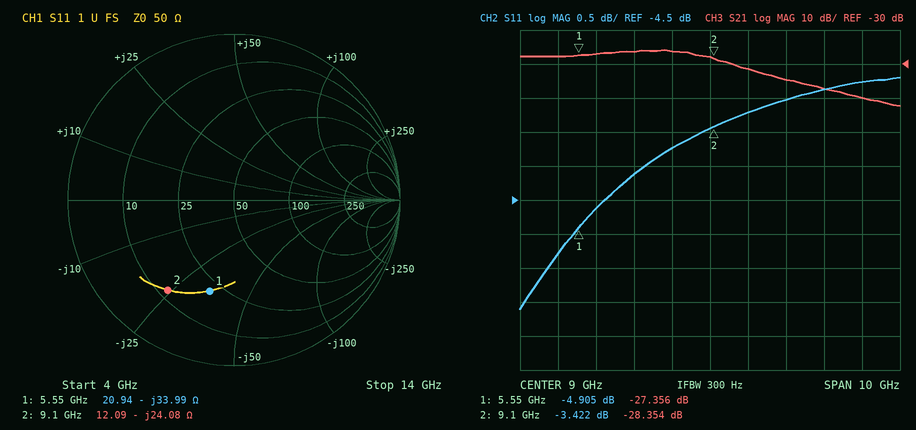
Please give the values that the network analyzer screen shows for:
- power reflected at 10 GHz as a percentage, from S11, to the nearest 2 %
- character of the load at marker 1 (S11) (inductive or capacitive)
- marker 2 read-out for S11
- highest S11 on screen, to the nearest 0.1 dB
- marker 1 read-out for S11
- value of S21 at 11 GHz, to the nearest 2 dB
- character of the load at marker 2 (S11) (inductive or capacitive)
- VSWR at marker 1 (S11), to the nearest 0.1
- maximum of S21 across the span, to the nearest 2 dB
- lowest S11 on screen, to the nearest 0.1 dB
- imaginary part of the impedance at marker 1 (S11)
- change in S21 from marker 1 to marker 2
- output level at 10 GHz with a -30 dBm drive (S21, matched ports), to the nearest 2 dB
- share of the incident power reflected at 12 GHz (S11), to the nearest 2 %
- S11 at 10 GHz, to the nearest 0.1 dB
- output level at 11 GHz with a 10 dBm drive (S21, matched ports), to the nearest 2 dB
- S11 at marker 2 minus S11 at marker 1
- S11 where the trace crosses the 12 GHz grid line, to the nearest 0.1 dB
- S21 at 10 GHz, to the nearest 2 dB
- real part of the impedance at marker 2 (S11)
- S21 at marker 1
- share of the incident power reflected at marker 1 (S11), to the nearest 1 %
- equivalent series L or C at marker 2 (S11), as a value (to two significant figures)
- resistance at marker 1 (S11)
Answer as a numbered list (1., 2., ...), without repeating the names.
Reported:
1. 48 %
2. capacitive
3. -3.422 dB
4. -2.7 dB
5. -4.905 dB
6. -34 dB
7. capacitive
8. 3.6
9. -26 dB
10. -6.1 dB
11. -33.99 Ω
12. -0.998 dB
13. -62 dBm
14. 52 %
15. -3.2 dB
16. -24 dBm
17. 1.483 dB
18. -2.9 dB
19. -32 dB
20. 12.09 Ω
21. -27.356 dB
22. 32 %
23. 730 fF
24. 20.94 Ω
